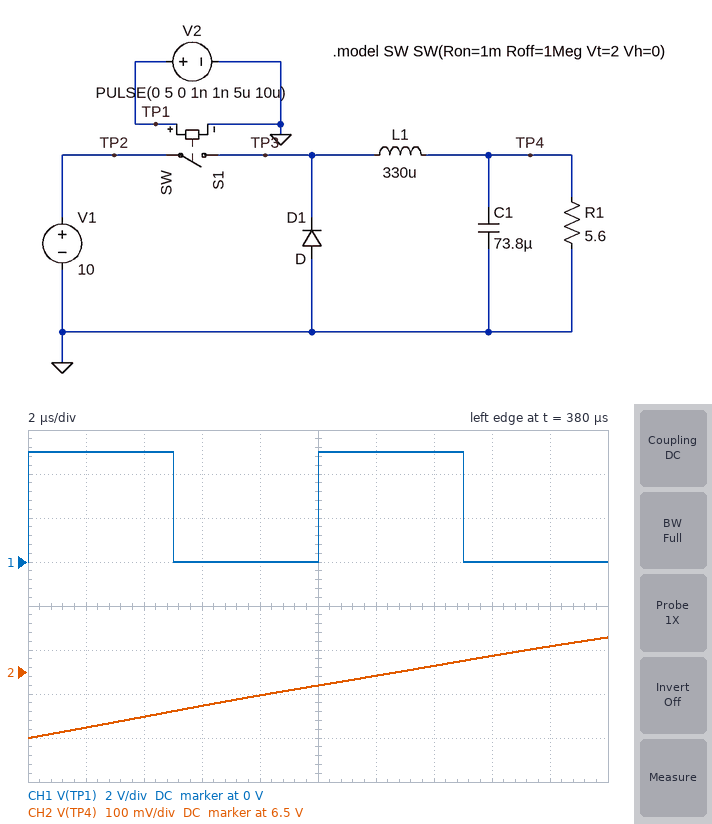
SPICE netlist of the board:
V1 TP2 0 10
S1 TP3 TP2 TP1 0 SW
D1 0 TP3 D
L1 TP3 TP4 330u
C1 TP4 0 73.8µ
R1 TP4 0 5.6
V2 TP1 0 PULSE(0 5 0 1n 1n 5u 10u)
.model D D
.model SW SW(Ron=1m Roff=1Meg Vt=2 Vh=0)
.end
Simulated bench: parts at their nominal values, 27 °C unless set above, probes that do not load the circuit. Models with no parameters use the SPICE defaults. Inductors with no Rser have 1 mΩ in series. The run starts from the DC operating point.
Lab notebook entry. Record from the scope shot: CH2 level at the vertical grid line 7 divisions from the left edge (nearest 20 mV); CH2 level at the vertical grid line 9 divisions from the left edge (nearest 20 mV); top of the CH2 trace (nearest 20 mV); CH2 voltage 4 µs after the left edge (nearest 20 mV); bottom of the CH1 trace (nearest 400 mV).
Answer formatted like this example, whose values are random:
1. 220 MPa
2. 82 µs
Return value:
1. 6.52 V
2. 6.56 V
3. 6.58 V
4. 6.40 V
5. 0 V
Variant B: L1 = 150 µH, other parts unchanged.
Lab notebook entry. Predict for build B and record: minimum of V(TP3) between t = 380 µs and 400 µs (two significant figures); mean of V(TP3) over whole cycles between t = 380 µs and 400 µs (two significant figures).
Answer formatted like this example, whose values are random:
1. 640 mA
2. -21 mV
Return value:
1. -810 mV
2. 5.1 V
